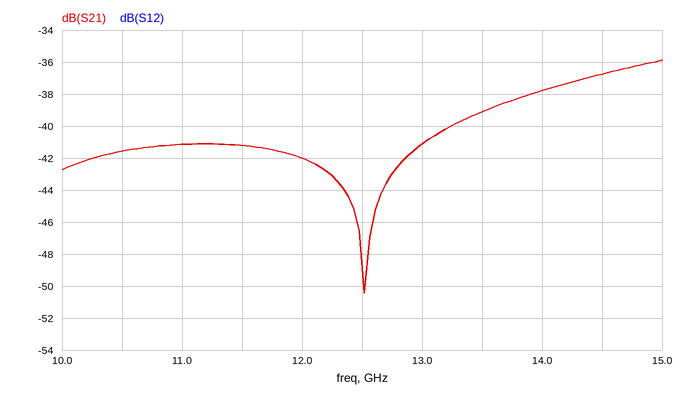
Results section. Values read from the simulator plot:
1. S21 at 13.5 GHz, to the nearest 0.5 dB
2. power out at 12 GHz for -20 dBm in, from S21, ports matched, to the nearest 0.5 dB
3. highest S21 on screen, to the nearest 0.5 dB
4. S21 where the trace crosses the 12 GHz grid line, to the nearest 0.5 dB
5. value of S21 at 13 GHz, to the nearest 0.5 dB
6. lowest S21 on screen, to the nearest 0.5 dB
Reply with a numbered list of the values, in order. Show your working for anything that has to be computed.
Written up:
1. -39.0 dB
2. -20 dBm + (-42.0 dB) = -62.0 dBm
3. -36.0 dB
4. -42.0 dB
5. -41.0 dB
6. -50.5 dB
